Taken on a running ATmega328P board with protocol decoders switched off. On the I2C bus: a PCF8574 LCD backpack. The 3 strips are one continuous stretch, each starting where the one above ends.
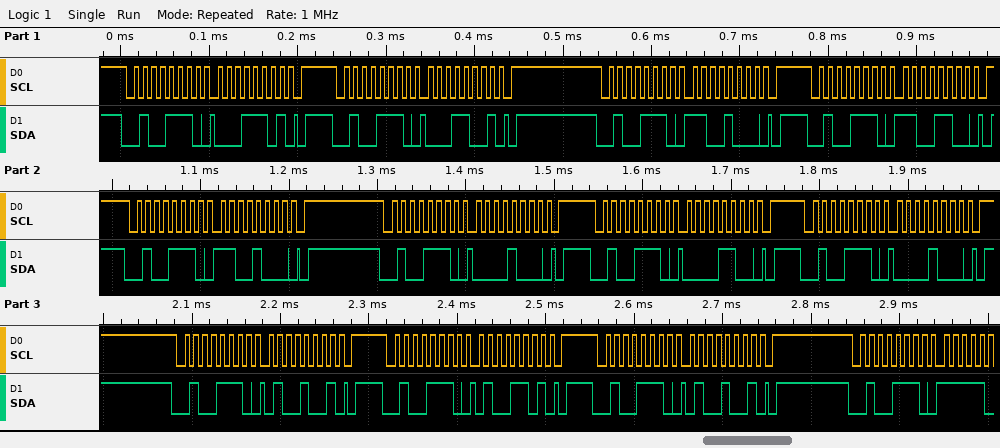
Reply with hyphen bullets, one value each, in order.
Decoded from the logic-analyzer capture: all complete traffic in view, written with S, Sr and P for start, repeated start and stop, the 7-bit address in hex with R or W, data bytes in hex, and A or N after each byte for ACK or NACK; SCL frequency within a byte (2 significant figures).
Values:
- S 27W A 1D A P S 27W A 19 A P S 27W A C8 A P S 27W A CC A P S 27W A C8 A P S 27W A 08 A P S 27W A 0C A P S 27W A 08 A P S 27W A 49 A P S 27W A 4D A P S 27W A 49 A P S 27W A
- 100 kHz
